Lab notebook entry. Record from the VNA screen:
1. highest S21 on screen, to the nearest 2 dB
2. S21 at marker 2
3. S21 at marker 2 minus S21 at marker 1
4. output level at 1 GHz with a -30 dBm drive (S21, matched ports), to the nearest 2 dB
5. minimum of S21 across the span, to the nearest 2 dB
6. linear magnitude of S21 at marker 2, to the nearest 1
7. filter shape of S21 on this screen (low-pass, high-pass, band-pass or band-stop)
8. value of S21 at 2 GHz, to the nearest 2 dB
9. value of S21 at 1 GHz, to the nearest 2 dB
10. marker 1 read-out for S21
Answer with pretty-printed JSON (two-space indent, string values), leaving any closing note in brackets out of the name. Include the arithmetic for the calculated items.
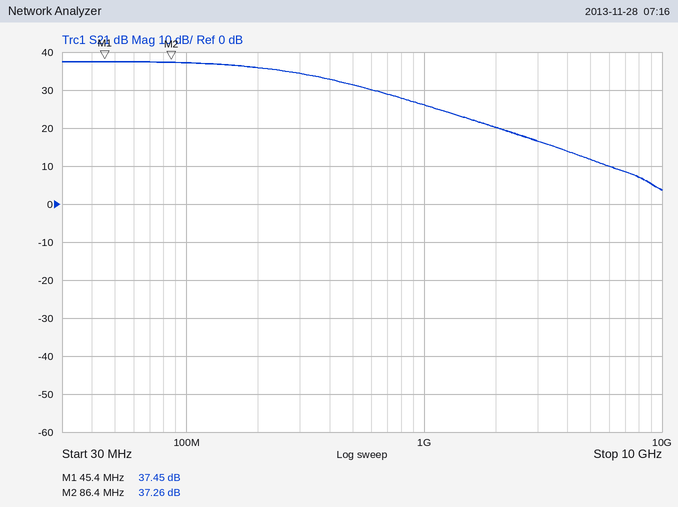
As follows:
{
  "highest S21 on screen, to the nearest 2 dB": "38 dB",
  "S21 at marker 2": "37.26 dB",
  "S21 at marker 2 minus S21 at marker 1": "37.26 − (37.45) = -0.19 dB",
  "output level at 1 GHz with a -30 dBm drive (S21, matched ports), to the nearest 2 dB": "-30 dBm + (26 dB) = -4 dBm",
  "minimum of S21 across the span, to the nearest 2 dB": "4 dB",
  "linear magnitude of S21 at marker 2, to the nearest 1": "10^(37.26/20) ≈ 73",
  "filter shape of S21 on this screen": "low-pass",
  "value of S21 at 2 GHz, to the nearest 2 dB": "20 dB",
  "value of S21 at 1 GHz, to the nearest 2 dB": "26 dB",
  "marker 1 read-out for S21": "37.45 dB"
}
